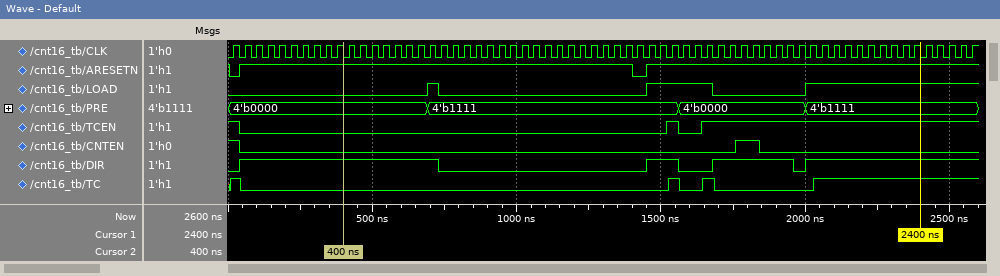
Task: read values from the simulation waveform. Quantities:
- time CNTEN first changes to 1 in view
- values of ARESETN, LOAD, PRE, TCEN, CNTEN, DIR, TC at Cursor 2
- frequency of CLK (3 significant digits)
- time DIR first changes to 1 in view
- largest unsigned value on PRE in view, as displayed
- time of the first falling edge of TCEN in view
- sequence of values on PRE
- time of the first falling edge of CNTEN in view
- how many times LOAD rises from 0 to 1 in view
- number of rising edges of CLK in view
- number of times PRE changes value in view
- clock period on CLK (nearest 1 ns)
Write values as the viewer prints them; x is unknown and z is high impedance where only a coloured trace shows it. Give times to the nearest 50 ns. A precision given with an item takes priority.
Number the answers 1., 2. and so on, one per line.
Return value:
1. 1750 ns
2. ARESETN=1, LOAD=0, PRE=4'b0000, TCEN=0, CNTEN=0, DIR=1, TC=0
3. 25.0 MHz
4. 50 ns
5. 4'b1111
6. 50 ns
7. 4'b0000, 4'b1111, 4'b0000, 4'b1111
8. 50 ns
9. 3
10. 65
11. 3
12. 40 ns
